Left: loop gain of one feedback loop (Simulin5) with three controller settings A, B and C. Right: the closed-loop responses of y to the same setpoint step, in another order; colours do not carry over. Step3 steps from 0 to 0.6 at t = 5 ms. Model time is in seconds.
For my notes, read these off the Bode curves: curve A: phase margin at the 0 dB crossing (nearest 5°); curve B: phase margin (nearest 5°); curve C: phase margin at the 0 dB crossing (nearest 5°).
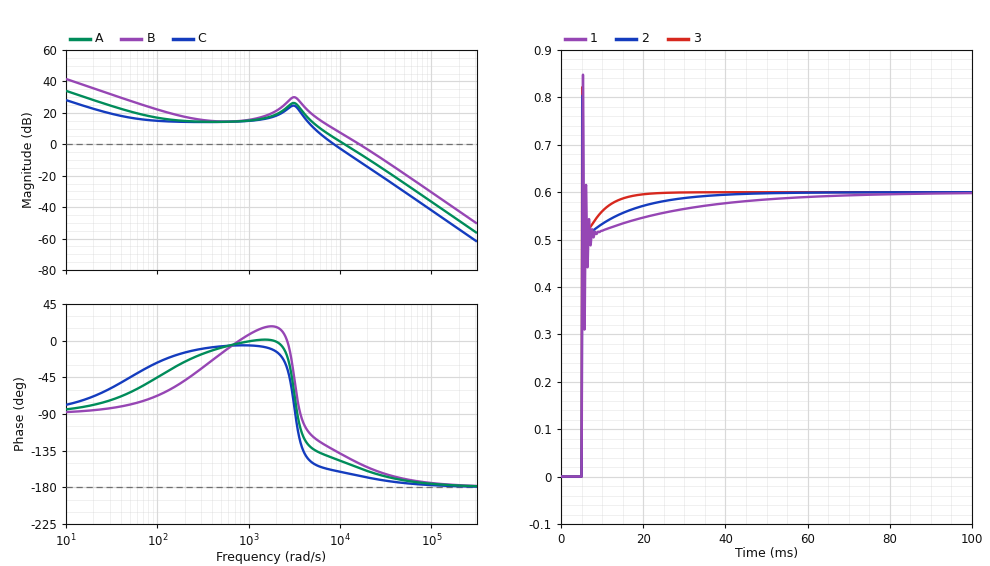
30°
30°
20°
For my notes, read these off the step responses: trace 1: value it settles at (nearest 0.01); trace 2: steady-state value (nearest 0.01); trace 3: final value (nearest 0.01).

0.60
0.60
0.60
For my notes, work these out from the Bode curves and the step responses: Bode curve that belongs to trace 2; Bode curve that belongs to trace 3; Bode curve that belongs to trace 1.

A
B
C
